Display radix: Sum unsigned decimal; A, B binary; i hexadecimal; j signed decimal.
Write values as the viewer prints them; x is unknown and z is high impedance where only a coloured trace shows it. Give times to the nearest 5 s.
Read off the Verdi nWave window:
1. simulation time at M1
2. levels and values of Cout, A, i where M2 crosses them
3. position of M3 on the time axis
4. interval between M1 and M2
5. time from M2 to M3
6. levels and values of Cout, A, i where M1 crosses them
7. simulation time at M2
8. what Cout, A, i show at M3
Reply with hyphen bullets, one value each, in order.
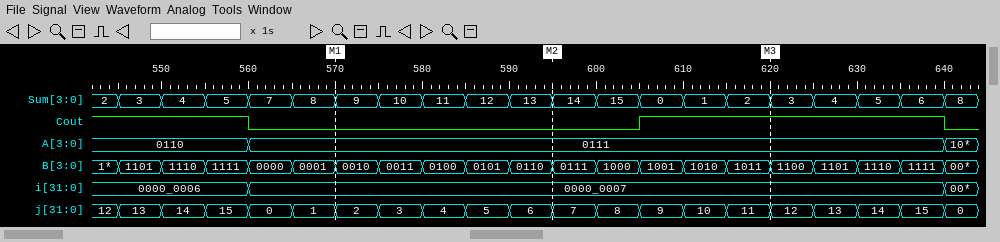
- 570 s
- Cout=0, A=0111, i=0000_0007
- 620 s
- 25 s
- 25 s
- Cout=0, A=0111, i=0000_0007
- 595 s
- Cout=1, A=0111, i=0000_0007
